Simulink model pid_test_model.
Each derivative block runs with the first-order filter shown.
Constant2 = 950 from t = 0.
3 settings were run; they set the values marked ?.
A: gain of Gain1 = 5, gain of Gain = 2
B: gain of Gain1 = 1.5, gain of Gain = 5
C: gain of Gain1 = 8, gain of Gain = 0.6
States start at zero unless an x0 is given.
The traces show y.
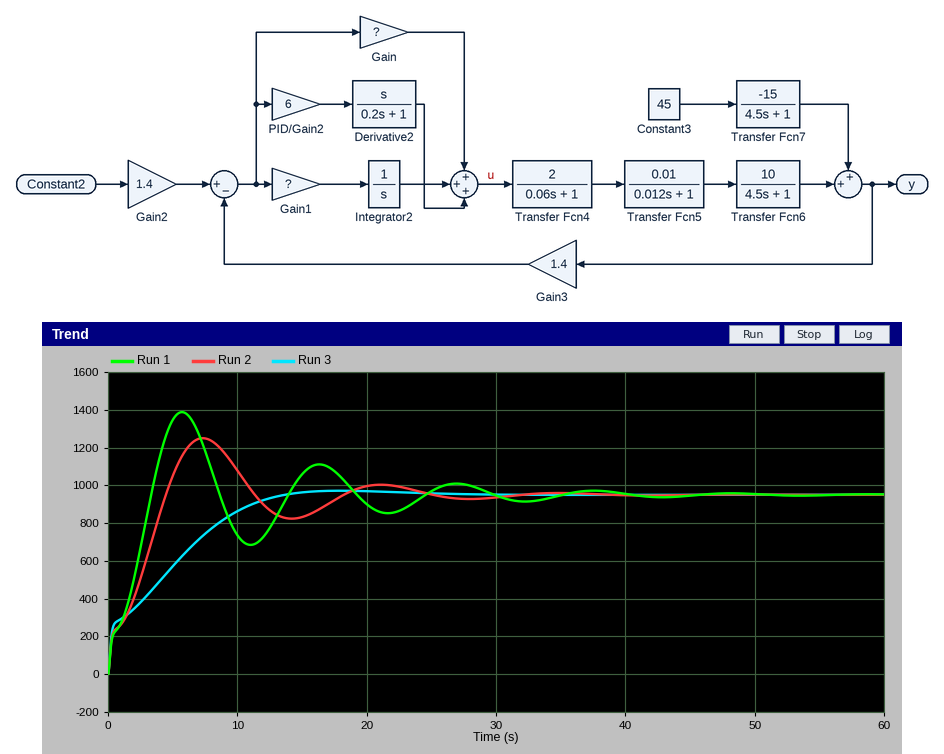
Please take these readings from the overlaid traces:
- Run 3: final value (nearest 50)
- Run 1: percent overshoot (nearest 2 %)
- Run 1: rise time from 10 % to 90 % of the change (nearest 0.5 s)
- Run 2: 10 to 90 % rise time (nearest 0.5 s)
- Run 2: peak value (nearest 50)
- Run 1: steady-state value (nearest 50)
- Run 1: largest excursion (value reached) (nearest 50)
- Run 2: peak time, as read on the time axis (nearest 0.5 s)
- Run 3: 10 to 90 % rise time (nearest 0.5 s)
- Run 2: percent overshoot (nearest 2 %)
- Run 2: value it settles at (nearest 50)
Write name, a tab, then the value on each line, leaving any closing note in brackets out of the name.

Run 3: final value	950
Run 1: percent overshoot	46 %
Run 1: rise time from 10 % to 90 % of the change	3.0 s
Run 2: 10 to 90 % rise time	4.0 s
Run 2: peak value	1250
Run 1: steady-state value	950
Run 1: largest excursion (value reached)	1400
Run 2: peak time, as read on the time axis	7.5 s
Run 3: 10 to 90 % rise time	9.5 s
Run 2: percent overshoot	32 %
Run 2: value it settles at	950
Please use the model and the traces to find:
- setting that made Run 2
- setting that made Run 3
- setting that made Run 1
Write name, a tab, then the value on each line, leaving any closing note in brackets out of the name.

setting that made Run 2	A
setting that made Run 3	B
setting that made Run 1	C
